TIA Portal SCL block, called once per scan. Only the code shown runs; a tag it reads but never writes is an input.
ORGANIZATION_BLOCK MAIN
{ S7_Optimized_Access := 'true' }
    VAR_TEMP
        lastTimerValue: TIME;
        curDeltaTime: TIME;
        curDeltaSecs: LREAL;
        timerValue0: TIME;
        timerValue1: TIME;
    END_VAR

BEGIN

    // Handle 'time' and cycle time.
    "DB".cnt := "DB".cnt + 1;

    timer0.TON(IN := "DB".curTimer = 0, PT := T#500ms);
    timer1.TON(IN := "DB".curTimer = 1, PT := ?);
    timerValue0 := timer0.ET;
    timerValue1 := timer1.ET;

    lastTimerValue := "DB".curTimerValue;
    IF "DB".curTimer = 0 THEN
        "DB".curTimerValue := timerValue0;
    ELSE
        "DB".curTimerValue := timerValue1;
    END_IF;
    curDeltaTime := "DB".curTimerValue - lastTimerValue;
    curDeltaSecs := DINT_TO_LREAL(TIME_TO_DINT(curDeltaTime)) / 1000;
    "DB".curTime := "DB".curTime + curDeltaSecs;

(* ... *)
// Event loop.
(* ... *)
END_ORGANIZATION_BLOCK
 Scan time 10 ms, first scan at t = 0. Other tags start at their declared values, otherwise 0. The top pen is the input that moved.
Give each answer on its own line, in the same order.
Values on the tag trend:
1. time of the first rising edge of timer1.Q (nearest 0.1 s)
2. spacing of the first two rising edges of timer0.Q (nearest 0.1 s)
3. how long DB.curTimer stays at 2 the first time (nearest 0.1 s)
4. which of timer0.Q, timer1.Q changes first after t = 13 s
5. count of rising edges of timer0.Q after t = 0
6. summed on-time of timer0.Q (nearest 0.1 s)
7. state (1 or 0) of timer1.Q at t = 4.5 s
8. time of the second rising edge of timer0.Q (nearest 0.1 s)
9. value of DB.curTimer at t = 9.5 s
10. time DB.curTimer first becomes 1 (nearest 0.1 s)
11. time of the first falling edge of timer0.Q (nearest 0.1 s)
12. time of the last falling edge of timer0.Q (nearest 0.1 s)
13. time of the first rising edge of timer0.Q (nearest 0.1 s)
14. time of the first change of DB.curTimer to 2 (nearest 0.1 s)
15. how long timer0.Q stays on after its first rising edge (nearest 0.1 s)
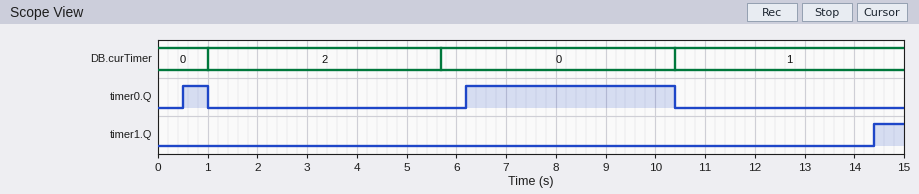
14.4 s
5.7 s
4.7 s
timer1.Q
2
4.7 s
0
6.2 s
0
10.4 s
1.0 s
10.4 s
0.5 s
1.0 s
0.5 s
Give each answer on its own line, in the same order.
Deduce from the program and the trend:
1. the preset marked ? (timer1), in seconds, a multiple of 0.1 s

4.0 s
